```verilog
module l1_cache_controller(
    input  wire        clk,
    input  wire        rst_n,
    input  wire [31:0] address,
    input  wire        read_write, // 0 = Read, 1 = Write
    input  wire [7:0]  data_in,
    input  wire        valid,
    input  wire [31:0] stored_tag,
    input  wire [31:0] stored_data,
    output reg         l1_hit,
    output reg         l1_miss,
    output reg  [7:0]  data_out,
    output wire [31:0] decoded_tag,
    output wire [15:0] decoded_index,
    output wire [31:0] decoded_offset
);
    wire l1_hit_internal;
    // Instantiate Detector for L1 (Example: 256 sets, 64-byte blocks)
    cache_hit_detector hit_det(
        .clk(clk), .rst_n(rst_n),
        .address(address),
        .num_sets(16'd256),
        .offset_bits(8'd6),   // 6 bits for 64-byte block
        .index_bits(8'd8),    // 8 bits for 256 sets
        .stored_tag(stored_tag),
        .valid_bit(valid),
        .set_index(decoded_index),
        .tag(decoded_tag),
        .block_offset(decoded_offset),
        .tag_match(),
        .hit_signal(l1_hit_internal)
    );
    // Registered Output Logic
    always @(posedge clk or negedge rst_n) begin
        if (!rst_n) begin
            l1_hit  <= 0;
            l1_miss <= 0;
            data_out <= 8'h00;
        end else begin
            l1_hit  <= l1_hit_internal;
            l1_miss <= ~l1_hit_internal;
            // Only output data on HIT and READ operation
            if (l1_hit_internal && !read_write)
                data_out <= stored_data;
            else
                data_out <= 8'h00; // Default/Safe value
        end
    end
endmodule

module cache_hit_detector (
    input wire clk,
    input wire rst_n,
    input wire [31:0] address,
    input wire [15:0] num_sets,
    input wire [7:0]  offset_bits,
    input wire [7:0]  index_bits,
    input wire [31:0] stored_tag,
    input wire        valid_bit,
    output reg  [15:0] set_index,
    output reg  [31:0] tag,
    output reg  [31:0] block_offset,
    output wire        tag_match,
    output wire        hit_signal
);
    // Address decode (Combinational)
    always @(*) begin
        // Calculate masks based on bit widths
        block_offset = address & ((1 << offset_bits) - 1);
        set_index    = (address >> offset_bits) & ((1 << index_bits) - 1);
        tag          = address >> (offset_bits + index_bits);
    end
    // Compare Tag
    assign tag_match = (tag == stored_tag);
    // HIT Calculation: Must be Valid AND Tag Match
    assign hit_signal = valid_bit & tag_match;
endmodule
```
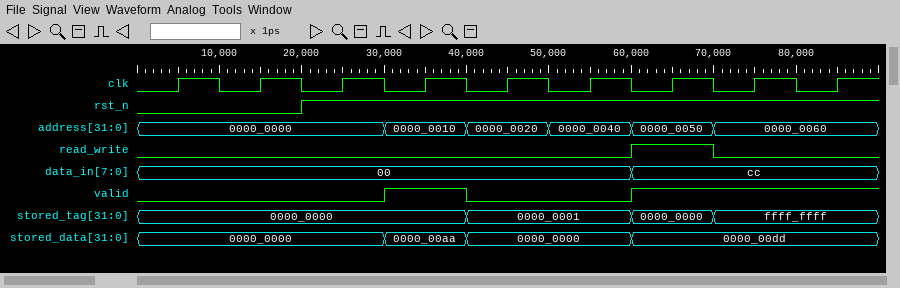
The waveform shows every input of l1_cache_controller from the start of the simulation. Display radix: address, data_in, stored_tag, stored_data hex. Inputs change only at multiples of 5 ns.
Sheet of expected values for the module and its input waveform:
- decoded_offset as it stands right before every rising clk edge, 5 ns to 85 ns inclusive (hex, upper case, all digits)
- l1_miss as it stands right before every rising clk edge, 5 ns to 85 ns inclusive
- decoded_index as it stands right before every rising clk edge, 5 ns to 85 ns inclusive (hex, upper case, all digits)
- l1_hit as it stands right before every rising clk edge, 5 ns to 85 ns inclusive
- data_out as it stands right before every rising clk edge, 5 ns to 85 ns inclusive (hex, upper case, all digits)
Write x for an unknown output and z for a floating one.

00000000, 00000000, 00000000, 00000010, 00000020, 00000000, 00000010, 00000020, 00000020
0 0 0 1 0 1 1 0 1
0000, 0000, 0000, 0000, 0000, 0001, 0001, 0001, 0001
0 0 0 0 1 0 0 1 0
00, 00, 00, 00, AA, 00, 00, 00, 00
